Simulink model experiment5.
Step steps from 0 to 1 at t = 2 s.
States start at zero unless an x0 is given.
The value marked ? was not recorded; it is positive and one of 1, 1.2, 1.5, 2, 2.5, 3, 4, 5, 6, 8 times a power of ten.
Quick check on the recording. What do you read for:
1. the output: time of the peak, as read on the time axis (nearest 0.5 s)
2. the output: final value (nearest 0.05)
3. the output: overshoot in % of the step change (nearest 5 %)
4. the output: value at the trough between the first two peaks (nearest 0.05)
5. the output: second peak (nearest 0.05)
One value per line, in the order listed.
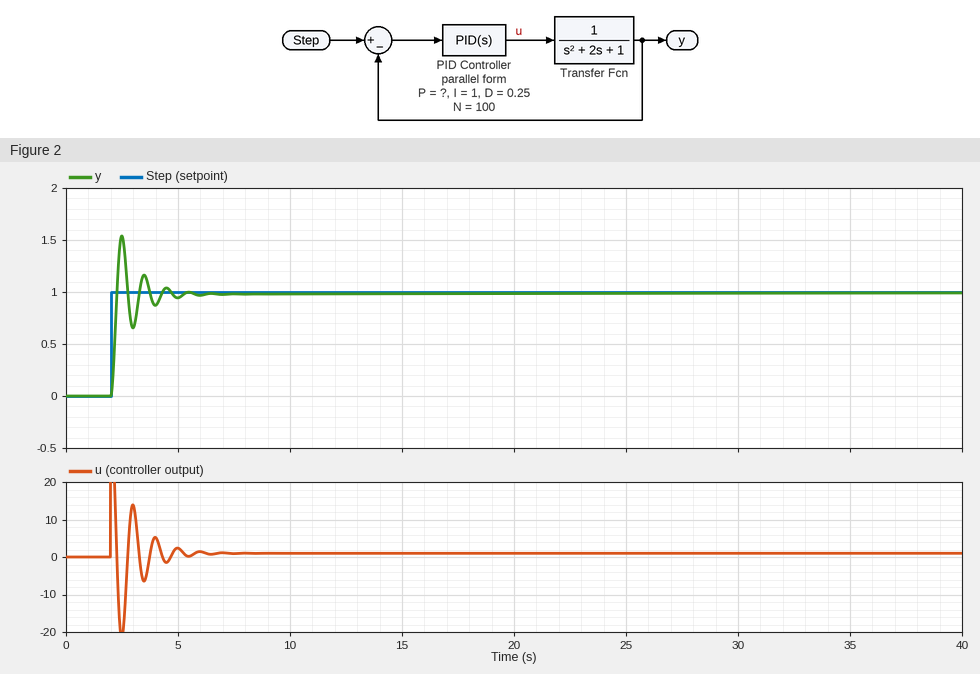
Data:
2.5 s
1.00
55 %
0.65
1.15
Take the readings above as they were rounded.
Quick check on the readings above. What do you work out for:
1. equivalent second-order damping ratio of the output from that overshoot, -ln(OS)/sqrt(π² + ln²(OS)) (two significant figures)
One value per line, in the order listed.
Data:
0.19
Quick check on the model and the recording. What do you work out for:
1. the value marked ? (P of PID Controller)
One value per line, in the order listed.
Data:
40
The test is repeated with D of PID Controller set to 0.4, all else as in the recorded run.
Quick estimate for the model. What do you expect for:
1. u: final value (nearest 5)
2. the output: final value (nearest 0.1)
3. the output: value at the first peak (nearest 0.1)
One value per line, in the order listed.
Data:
0
1.0
1.5
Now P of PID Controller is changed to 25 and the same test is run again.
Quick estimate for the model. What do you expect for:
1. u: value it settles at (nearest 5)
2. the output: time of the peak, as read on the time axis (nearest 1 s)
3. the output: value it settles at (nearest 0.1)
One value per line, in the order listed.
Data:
0
3 s
1.0
